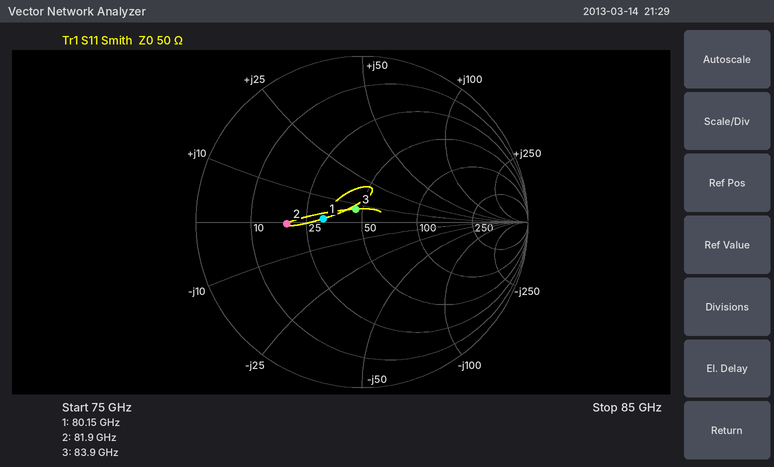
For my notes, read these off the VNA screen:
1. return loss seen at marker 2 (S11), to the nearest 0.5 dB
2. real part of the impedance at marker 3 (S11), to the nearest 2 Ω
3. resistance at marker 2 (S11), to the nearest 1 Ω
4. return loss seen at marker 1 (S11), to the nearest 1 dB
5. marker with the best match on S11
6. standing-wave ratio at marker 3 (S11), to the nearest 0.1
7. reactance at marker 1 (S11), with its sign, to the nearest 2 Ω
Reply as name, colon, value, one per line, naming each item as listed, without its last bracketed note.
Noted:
return loss seen at marker 2 (S11), to the nearest 0.5 dB: 7.0 dB
real part of the impedance at marker 3 (S11), to the nearest 2 Ω: 46 Ω
resistance at marker 2 (S11), to the nearest 1 Ω: 19 Ω
return loss seen at marker 1 (S11), to the nearest 1 dB: 13 dB
marker with the best match on S11: marker 3
standing-wave ratio at marker 3 (S11), to the nearest 0.1: 1.2
reactance at marker 1 (S11), with its sign, to the nearest 2 Ω: +2 Ω
